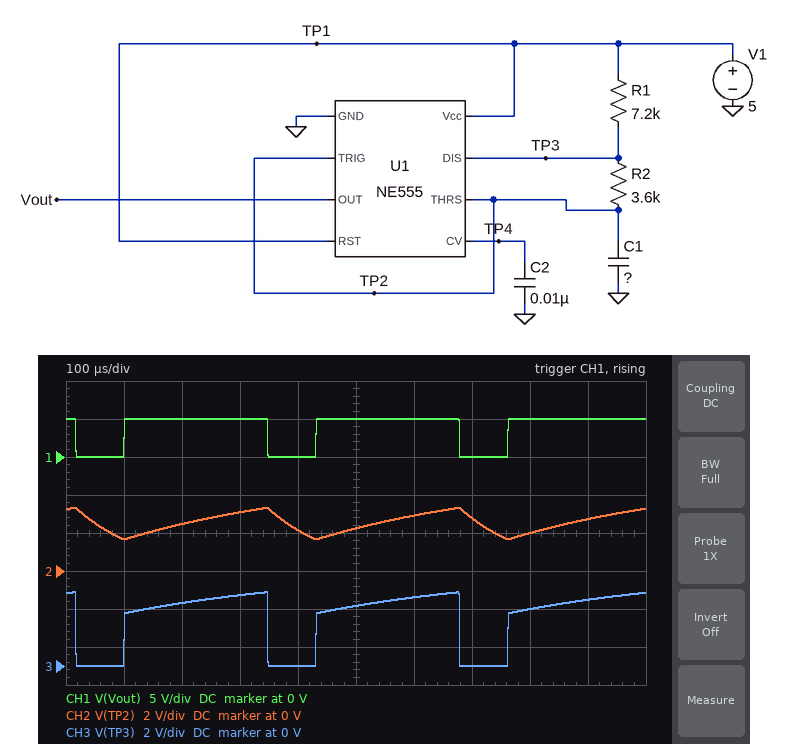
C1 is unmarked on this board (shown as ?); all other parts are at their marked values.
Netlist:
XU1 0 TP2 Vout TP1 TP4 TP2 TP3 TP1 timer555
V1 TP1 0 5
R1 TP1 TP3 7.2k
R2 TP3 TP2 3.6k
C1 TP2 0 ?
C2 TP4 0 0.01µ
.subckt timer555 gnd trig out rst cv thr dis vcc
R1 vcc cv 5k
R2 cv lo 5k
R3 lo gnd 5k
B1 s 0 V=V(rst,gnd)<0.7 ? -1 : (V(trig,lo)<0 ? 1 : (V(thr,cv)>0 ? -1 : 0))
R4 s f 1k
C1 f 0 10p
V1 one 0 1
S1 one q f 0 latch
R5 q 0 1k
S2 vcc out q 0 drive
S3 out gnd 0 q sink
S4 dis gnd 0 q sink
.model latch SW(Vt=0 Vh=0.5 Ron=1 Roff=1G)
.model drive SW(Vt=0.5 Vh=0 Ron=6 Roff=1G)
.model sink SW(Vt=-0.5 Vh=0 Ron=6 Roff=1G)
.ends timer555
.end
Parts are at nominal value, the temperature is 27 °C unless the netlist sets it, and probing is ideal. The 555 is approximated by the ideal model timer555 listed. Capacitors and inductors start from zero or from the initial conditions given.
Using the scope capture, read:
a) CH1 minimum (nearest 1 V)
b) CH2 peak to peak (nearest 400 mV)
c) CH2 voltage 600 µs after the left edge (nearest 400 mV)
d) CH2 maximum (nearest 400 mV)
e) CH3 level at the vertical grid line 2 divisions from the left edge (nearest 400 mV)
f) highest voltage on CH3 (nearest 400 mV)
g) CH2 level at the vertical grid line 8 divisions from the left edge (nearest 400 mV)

0 V
1.6 V
2.8 V
3.2 V
3.2 V
4.0 V
2.0 V
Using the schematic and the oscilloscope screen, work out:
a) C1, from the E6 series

33 nF
